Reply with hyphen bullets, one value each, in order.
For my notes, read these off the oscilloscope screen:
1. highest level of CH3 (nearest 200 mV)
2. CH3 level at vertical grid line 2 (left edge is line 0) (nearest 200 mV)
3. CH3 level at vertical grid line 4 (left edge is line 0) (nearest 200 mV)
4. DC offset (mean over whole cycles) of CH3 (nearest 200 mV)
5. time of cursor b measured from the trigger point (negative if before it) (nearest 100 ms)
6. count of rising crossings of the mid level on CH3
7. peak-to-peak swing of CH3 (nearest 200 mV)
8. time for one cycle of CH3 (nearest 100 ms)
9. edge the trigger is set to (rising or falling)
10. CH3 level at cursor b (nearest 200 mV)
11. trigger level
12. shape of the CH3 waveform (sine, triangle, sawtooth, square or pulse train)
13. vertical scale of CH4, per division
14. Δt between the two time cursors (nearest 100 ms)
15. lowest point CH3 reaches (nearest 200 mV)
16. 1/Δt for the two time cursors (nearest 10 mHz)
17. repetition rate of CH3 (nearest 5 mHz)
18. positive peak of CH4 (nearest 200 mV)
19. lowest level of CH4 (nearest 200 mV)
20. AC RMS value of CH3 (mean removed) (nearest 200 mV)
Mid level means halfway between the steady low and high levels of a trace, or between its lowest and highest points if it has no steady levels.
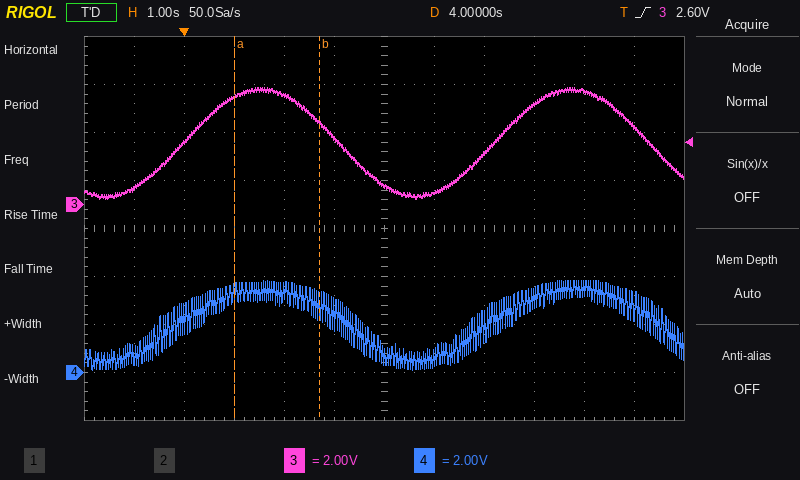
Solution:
- 4.8 V
- 2.6 V
- 4.6 V
- 2.6 V
- +2.7 s
- 2
- 4.6 V
- 6.2 s
- rising
- 3.4 V
- 2.60 V
- sine
- 2 V
- 1.7 s
- 200 mV
- 590 mHz
- 160 mHz
- 3.8 V
- 200 mV
- 1.6 V
